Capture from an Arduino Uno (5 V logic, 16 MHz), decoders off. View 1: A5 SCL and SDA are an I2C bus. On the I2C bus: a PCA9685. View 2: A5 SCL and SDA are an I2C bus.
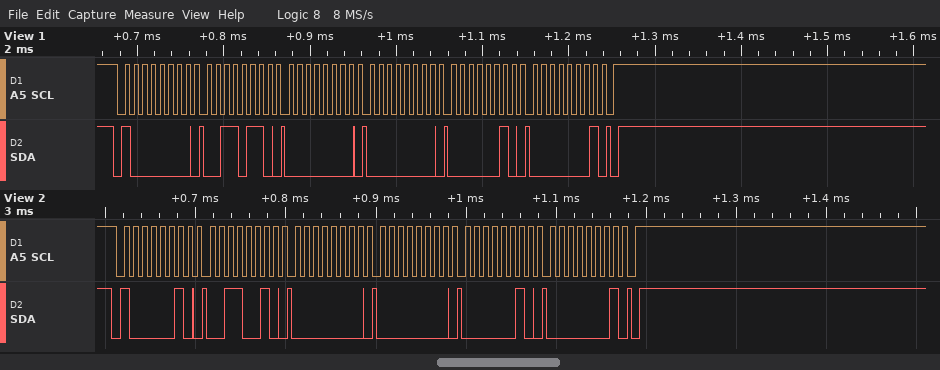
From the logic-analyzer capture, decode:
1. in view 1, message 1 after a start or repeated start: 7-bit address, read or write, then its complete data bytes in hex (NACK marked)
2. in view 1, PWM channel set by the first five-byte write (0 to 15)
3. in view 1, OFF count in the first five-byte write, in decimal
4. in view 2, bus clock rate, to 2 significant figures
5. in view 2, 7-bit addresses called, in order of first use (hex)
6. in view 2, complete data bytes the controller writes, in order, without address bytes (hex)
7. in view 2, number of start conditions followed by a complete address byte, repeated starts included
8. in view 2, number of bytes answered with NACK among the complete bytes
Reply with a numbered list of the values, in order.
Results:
1. 0x40 write: 36 00 00 02 01
2. 12
3. 258
4. 100 kHz
5. 0x41
6. 32 00 00 02 01
7. 1
8. 0
